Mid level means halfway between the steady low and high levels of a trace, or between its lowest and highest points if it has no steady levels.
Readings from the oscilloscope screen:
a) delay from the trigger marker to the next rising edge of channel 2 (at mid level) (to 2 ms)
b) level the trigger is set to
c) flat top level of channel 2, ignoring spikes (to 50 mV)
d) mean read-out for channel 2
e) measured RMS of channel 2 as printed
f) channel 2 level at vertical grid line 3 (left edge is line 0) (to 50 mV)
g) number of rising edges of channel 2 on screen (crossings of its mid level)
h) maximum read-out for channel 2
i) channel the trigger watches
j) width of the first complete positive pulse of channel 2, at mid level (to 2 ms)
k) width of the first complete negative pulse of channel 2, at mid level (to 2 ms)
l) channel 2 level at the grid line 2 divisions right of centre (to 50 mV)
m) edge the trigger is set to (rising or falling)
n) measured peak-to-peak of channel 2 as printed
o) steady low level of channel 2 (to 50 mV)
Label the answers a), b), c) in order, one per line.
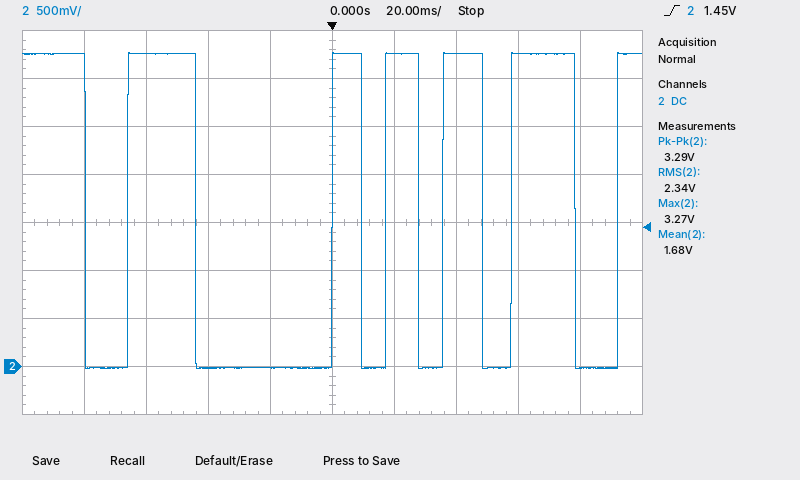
a) 18 ms
b) 1.45 V
c) 3.25 V
d) 1.68 V
e) 2.34 V
f) 0 mV
g) 6
h) 3.27 V
i) channel 2
j) 22 ms
k) 14 ms
l) 3.25 V
m) rising
n) 3.29 V
o) 0 mV
